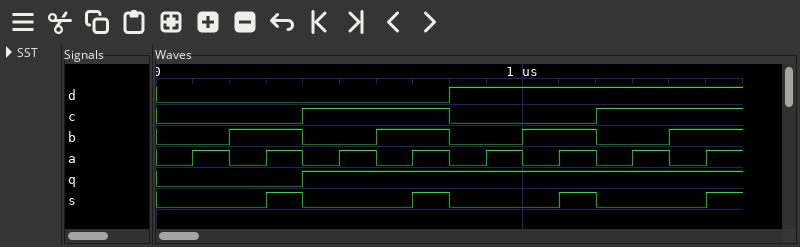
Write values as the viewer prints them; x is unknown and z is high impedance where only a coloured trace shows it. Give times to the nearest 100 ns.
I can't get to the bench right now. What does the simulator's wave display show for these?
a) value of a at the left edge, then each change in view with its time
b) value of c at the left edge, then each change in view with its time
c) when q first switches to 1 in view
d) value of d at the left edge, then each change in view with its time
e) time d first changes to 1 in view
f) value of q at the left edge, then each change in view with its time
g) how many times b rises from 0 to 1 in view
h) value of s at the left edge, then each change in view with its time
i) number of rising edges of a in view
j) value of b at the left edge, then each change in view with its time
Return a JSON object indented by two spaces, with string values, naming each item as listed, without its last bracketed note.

{
  "value of a at the left edge, then each change in view with its time": "0, 1 at 100 ns, 0 at 200 ns, 1 at 300 ns, 0 at 400 ns, 1 at 500 ns, 0 at 600 ns, 1 at 700 ns, 0 at 800 ns, 1 at 900 ns, 0 at 1000 ns, 1 at 1100 ns, 0 at 1200 ns, 1 at 1300 ns, 0 at 1400 ns, 1 at 1500 ns",
  "value of c at the left edge, then each change in view with its time": "0, 1 at 400 ns, 0 at 800 ns, 1 at 1200 ns",
  "when q first switches to 1 in view": "400 ns",
  "value of d at the left edge, then each change in view with its time": "0, 1 at 800 ns",
  "time d first changes to 1 in view": "800 ns",
  "value of q at the left edge, then each change in view with its time": "0, 1 at 400 ns",
  "how many times b rises from 0 to 1 in view": "4",
  "value of s at the left edge, then each change in view with its time": "0, 1 at 300 ns, 0 at 400 ns, 1 at 700 ns, 0 at 800 ns, 1 at 1100 ns, 0 at 1200 ns, 1 at 1500 ns",
  "number of rising edges of a in view": "8",
  "value of b at the left edge, then each change in view with its time": "0, 1 at 200 ns, 0 at 400 ns, 1 at 600 ns, 0 at 800 ns, 1 at 1000 ns, 0 at 1200 ns, 1 at 1400 ns"
}
